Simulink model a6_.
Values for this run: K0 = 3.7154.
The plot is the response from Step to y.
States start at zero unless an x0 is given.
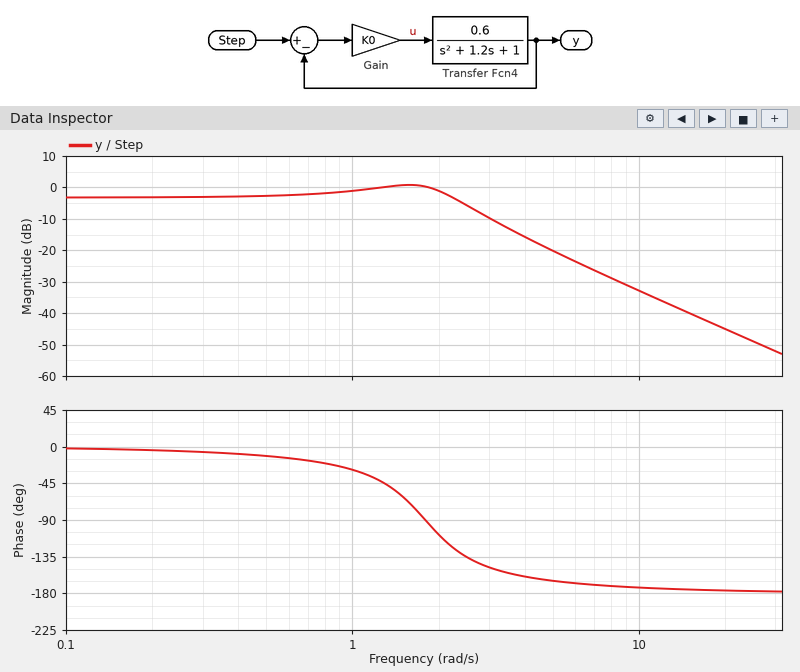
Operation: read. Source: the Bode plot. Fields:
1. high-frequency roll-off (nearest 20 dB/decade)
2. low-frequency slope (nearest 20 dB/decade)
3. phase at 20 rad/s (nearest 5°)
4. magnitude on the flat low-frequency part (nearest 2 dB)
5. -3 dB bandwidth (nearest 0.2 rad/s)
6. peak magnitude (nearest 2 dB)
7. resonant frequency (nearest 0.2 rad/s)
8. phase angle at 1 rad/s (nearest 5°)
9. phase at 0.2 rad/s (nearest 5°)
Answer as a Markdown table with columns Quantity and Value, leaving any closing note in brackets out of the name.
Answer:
| Quantity | Value |
|---|---|
| high-frequency roll-off | -40 dB/decade |
| low-frequency slope | 0 dB/decade |
| phase at 20 rad/s | -175° |
| magnitude on the flat low-frequency part | -4 dB |
| -3 dB bandwidth | 2.6 rad/s |
| peak magnitude | 0 dB |
| resonant frequency | 1.6 rad/s |
| phase angle at 1 rad/s | -30° |
| phase at 0.2 rad/s | -5° |
